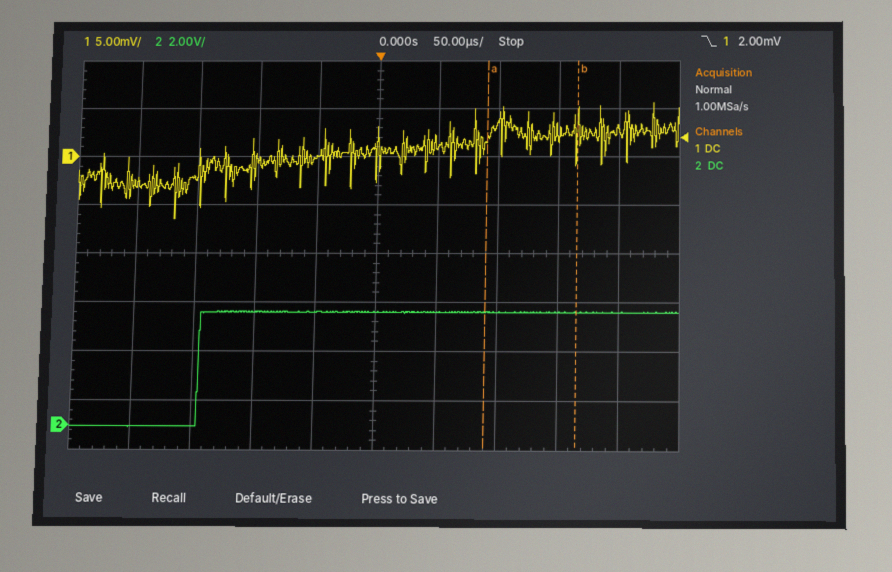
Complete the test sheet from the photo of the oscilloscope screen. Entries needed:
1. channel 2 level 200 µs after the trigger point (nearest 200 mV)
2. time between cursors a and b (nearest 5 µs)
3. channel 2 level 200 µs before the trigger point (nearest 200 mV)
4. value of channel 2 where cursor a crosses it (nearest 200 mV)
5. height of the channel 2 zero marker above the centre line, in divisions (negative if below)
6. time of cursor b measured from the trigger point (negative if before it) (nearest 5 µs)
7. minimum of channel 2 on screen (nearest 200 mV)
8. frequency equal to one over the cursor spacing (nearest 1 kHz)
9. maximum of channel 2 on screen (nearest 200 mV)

4.6 V
75 µs
0.0 V
4.6 V
-3.5 div
+165 µs
0.0 V
13 kHz
4.6 V
